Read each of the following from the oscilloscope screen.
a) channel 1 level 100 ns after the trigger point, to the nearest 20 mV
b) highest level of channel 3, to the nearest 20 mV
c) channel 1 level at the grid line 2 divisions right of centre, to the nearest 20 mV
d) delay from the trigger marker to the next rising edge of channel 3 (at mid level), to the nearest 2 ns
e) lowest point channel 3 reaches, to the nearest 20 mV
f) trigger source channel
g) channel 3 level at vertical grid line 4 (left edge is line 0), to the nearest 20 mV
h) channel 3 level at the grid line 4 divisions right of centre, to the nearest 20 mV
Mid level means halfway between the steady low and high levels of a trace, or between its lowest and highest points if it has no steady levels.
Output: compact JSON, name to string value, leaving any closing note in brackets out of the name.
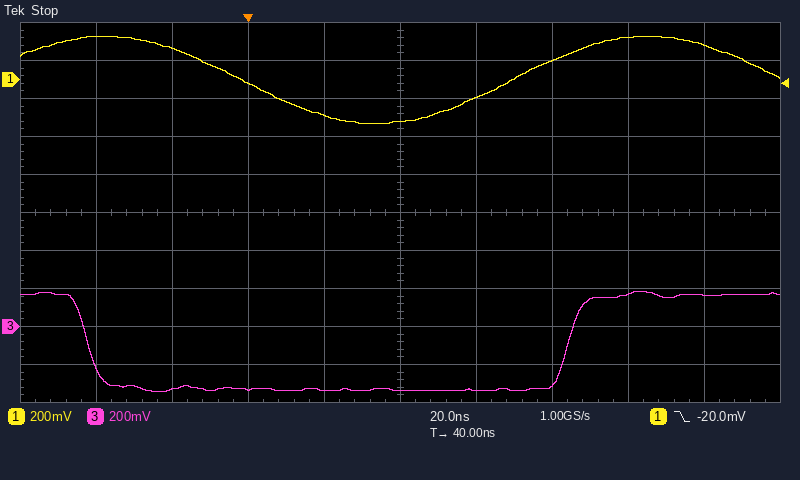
{"channel 1 level 100 ns after the trigger point, to the nearest 20 mV": "220 mV", "highest level of channel 3, to the nearest 20 mV": "180 mV", "channel 1 level at the grid line 2 divisions right of centre, to the nearest 20 mV": "100 mV", "delay from the trigger marker to the next rising edge of channel 3 (at mid level), to the nearest 2 ns": "84 ns", "lowest point channel 3 reaches, to the nearest 20 mV": "-340 mV", "trigger source channel": "channel 1", "channel 3 level at vertical grid line 4 (left edge is line 0), to the nearest 20 mV": "-340 mV", "channel 3 level at the grid line 4 divisions right of centre, to the nearest 20 mV": "160 mV"}
